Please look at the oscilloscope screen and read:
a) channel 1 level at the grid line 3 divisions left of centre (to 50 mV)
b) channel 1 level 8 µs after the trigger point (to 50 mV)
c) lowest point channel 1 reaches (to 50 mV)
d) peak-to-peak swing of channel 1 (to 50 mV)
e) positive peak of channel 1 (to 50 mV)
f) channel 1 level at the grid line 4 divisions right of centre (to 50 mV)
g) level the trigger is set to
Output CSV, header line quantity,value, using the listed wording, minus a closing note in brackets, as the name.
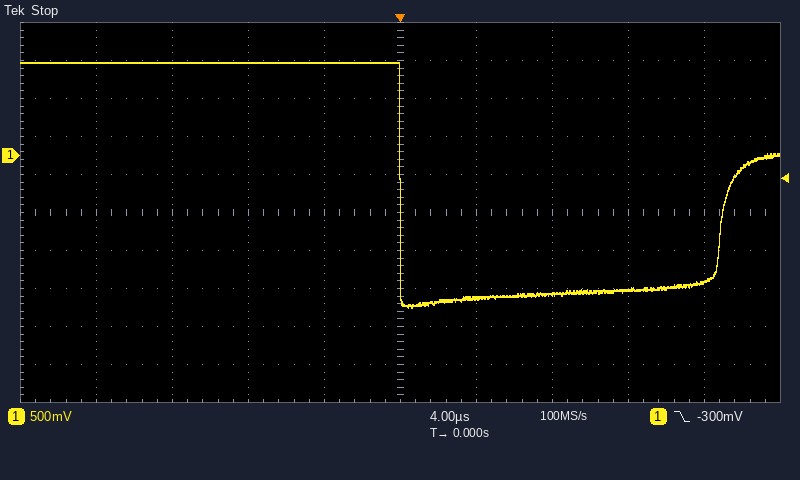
quantity,value
channel 1 level at the grid line 3 divisions left of centre,1.20 V
channel 1 level 8 µs after the trigger point,-1.80 V
lowest point channel 1 reaches,-2.00 V
peak-to-peak swing of channel 1,3.20 V
positive peak of channel 1,1.20 V
channel 1 level at the grid line 4 divisions right of centre,-1.65 V
level the trigger is set to,-300 mV
